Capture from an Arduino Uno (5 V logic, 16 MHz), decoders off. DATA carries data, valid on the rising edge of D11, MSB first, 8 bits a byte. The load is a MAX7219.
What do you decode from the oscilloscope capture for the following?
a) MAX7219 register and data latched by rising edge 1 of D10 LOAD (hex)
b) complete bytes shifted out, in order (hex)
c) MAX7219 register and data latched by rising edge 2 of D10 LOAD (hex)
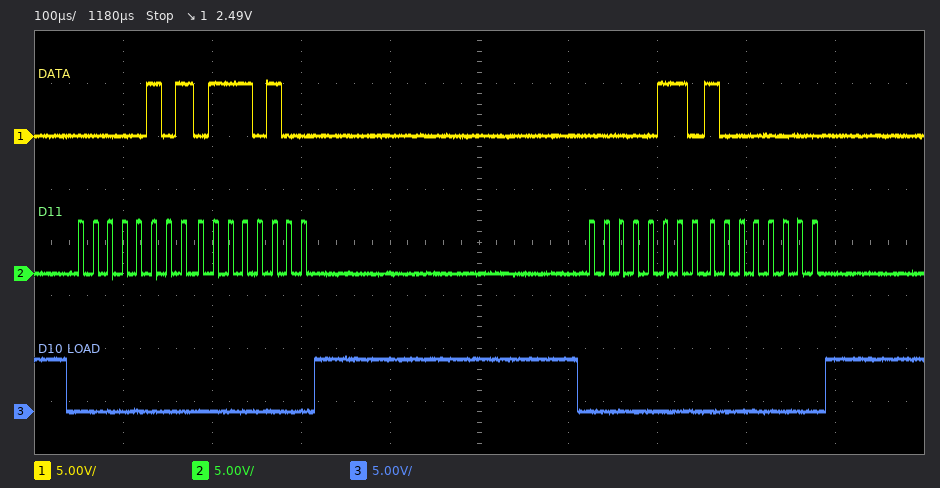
register 0x5, data 0x74
0x05 0x74 0x06 0x80
register 0x6, data 0x80
